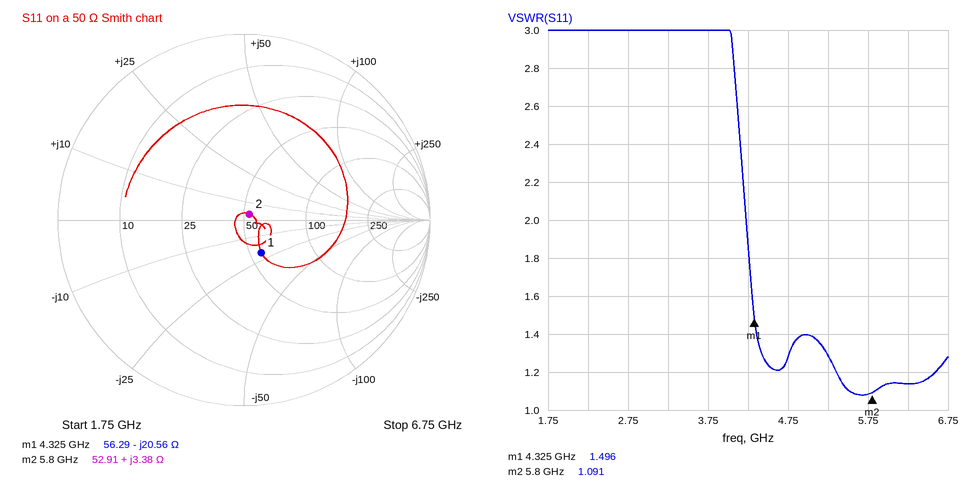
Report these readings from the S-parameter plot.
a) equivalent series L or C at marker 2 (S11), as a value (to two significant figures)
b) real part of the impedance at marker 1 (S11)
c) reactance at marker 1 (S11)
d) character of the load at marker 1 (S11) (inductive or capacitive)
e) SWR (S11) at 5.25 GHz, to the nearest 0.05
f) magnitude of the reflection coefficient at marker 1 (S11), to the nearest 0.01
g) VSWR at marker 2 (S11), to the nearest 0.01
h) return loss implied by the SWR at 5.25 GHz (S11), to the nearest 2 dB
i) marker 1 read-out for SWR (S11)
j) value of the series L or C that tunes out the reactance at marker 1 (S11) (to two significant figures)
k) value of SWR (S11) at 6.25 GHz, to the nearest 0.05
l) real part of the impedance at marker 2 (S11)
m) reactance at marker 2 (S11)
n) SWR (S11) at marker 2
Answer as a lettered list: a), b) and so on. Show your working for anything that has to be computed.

a) L = 3.38 Ω/(2π × 5.8 GHz) ≈ 93 pH
b) 56.29 Ω
c) -20.56 Ω
d) capacitive
e) 1.30
f) 0.20
g) 1.09
h) −20 log10((1.3 − 1)/(1.3 + 1)) ≈ 18 dB
i) 1.496
j) L = 20.56 Ω/(2π × 4.325 GHz) ≈ 757 pH, so 760 pH to two significant figures
k) 1.15
l) 52.91 Ω
m) +3.38 Ω
n) 1.091
